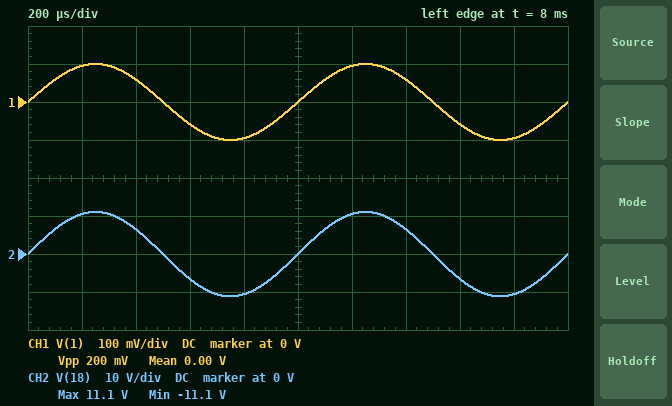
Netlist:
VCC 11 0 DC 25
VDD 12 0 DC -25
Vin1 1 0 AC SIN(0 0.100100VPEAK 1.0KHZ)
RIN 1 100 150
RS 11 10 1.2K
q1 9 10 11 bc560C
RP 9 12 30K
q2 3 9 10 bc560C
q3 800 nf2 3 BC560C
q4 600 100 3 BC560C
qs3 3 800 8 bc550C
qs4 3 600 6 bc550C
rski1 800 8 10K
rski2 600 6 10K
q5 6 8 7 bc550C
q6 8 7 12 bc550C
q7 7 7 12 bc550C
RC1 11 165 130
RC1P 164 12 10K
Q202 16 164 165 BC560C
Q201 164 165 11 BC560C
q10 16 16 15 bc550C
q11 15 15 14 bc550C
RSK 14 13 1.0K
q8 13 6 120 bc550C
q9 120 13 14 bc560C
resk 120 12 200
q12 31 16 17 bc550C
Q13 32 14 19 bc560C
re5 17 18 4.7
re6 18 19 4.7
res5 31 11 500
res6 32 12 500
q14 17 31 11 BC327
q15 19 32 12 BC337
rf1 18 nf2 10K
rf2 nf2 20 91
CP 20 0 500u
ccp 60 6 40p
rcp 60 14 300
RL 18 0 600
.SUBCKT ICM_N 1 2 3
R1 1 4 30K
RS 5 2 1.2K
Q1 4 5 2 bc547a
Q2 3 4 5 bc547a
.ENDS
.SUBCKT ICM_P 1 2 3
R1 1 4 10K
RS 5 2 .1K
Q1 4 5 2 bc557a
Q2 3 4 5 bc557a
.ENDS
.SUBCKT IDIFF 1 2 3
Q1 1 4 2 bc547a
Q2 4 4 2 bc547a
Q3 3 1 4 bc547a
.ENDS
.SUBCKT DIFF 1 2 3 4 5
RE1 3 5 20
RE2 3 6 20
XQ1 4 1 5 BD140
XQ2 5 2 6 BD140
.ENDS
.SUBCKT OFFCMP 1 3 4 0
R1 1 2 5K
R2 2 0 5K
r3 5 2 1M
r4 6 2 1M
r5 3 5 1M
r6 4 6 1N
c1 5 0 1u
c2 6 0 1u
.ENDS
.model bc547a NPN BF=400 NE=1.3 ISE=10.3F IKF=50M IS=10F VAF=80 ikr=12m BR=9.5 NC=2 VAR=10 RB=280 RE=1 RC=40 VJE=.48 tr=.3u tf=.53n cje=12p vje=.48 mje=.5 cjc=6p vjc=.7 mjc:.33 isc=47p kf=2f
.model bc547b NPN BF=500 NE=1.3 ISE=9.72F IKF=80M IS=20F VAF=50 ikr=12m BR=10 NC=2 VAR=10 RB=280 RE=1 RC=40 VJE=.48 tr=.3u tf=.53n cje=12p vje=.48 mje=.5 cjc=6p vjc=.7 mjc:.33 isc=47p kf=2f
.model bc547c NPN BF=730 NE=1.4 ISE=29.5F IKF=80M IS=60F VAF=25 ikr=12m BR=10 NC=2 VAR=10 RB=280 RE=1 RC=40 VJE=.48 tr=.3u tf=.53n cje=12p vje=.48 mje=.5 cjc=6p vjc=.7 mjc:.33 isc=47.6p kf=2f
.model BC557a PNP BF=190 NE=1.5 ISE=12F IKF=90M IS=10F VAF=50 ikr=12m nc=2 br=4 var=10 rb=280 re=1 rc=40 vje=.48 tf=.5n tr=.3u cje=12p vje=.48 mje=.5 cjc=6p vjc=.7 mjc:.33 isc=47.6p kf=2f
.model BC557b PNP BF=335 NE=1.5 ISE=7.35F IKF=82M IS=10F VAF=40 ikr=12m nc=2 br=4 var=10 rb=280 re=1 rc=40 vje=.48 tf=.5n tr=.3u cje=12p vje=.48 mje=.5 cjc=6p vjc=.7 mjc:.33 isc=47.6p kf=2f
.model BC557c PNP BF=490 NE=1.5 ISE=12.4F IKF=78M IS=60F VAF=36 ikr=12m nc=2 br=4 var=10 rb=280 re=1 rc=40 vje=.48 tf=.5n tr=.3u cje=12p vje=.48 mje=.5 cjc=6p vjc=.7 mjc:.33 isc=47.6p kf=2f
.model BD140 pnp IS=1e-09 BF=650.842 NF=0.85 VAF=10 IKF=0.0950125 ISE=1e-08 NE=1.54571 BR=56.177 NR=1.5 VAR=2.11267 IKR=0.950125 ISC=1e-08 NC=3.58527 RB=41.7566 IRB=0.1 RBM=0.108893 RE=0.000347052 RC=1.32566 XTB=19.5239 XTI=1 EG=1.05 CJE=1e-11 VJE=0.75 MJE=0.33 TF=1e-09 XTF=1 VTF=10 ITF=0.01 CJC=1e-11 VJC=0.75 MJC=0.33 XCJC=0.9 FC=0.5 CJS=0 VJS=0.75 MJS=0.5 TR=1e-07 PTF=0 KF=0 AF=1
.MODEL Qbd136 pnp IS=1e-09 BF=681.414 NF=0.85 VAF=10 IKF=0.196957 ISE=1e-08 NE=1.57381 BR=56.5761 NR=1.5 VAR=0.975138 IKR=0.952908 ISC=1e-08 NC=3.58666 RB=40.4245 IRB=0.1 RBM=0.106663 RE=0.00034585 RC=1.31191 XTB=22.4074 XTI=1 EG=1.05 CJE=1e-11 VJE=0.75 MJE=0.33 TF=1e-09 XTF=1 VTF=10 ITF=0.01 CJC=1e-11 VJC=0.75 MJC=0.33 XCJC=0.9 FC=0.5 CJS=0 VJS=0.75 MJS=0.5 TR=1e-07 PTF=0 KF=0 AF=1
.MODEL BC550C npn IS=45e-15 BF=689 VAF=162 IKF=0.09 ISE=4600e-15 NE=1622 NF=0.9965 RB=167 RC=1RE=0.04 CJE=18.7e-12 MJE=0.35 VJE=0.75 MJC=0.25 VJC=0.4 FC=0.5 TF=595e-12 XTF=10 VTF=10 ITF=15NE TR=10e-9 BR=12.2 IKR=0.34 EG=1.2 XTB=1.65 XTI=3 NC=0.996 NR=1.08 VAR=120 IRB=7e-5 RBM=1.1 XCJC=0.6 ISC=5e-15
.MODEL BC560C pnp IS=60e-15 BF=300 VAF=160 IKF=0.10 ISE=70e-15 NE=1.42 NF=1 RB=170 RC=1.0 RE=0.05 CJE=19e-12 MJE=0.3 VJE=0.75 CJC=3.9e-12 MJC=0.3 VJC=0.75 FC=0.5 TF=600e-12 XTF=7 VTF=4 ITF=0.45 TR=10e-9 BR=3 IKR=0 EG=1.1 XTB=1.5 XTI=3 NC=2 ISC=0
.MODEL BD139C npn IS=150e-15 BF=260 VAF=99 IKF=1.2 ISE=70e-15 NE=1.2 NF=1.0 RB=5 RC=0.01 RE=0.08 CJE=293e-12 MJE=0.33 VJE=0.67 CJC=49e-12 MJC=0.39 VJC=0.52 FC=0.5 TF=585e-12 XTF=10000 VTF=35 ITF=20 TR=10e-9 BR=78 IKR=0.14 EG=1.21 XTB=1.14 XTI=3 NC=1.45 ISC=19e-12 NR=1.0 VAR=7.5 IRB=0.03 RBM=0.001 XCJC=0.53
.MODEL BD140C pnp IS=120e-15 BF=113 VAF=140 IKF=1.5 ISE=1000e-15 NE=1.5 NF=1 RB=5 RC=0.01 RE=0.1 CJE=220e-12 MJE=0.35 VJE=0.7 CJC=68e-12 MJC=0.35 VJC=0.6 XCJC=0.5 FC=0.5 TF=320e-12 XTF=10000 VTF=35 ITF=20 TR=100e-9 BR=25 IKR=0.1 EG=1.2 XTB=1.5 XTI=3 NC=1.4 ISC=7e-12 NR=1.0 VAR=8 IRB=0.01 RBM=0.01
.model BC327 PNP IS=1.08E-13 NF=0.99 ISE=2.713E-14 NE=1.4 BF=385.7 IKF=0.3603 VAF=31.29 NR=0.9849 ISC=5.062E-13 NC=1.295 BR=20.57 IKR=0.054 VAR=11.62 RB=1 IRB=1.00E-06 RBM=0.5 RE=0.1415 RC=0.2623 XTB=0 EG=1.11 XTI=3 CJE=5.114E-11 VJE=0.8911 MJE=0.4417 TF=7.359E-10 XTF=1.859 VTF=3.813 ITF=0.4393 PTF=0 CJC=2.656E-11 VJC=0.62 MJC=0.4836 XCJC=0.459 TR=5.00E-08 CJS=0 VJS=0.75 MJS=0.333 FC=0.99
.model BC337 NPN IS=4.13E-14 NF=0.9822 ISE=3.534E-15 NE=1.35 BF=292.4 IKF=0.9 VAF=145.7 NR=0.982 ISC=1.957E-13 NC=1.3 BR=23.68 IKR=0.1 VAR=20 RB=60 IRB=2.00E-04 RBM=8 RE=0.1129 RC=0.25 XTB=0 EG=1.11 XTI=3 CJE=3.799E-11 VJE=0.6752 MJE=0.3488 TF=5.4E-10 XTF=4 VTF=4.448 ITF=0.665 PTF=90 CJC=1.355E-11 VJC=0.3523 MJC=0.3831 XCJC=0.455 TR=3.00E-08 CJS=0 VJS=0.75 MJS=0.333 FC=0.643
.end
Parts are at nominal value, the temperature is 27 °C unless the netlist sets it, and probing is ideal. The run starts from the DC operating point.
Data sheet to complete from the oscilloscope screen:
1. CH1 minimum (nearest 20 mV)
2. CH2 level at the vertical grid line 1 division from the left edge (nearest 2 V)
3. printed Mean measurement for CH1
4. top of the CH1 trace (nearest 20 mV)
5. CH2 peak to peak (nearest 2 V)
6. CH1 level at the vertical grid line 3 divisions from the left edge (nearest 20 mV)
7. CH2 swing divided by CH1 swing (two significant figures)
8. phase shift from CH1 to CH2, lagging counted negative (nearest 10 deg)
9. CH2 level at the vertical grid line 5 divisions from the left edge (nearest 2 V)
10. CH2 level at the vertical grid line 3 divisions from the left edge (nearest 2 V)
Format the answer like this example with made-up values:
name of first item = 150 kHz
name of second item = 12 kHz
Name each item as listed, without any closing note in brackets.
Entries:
CH1 minimum = -100 mV
CH2 level at the vertical grid line 1 division from the left edge = 10 V
printed Mean measurement for CH1 = 0.00 V
top of the CH1 trace = 100 mV
CH2 peak to peak = 22 V
CH1 level at the vertical grid line 3 divisions from the left edge = -60 mV
CH2 swing divided by CH1 swing = 110
phase shift from CH1 to CH2, lagging counted negative = 0 deg
CH2 level at the vertical grid line 5 divisions from the left edge = 0 V
CH2 level at the vertical grid line 3 divisions from the left edge = -6 V
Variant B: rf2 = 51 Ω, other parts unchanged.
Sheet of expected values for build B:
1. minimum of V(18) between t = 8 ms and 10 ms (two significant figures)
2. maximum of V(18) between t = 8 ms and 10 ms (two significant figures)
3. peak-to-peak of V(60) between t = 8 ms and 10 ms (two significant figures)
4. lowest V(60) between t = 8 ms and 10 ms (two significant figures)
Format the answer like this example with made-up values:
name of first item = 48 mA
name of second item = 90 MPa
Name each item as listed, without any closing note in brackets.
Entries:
minimum of V(18) between t = 8 ms and 10 ms = -20 V
maximum of V(18) between t = 8 ms and 10 ms = 20 V
peak-to-peak of V(60) between t = 8 ms and 10 ms = 40 V
lowest V(60) between t = 8 ms and 10 ms = -21 V
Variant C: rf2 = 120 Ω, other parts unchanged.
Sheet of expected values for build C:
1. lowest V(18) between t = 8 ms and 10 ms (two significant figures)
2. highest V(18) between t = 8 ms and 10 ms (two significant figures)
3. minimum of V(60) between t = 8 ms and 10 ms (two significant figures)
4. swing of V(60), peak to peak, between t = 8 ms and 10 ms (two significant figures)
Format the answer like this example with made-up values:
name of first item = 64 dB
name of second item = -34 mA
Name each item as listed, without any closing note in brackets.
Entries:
lowest V(18) between t = 8 ms and 10 ms = -8.5 V
highest V(18) between t = 8 ms and 10 ms = 8.4 V
minimum of V(60) between t = 8 ms and 10 ms = -9.2 V
swing of V(60), peak to peak, between t = 8 ms and 10 ms = 17 V
